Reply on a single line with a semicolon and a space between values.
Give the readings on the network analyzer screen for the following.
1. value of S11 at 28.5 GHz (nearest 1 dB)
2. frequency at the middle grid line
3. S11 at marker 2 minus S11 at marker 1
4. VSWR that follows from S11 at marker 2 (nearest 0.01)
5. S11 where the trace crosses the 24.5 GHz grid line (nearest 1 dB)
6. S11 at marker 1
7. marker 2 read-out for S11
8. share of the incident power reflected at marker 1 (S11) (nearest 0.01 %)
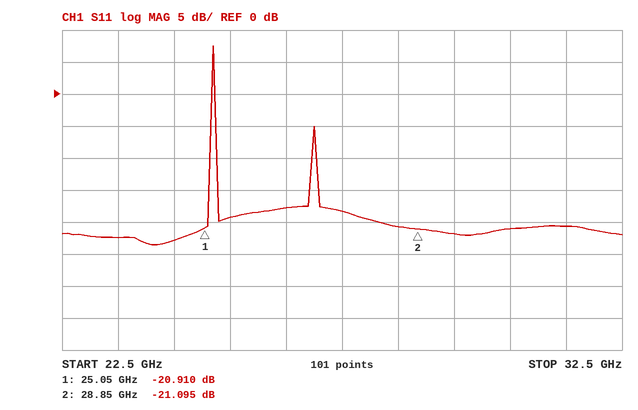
-21 dB; 27.5 GHz; -0.185 dB; 1.19; -23 dB; -20.910 dB; -21.095 dB; 0.81 %
